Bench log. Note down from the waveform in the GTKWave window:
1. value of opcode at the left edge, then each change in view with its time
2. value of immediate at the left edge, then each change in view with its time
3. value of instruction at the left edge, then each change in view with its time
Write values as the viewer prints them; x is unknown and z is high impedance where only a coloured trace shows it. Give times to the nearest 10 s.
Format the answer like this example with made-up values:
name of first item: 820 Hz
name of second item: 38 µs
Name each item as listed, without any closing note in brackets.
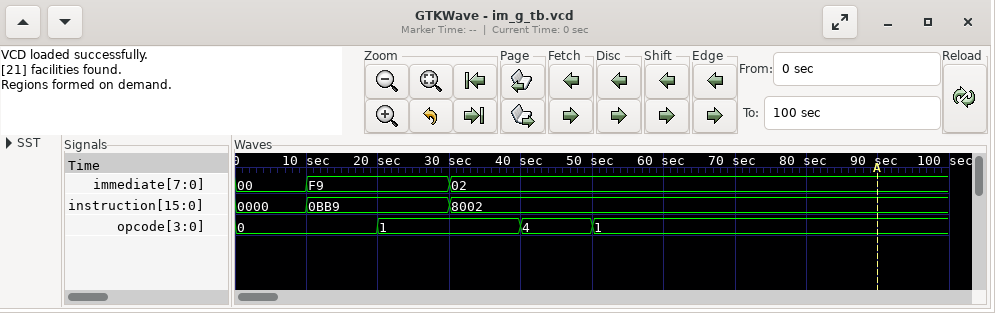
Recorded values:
value of opcode at the left edge, then each change in view with its time: 0, 1 at 20 s, 4 at 40 s, 1 at 50 s
value of immediate at the left edge, then each change in view with its time: 00, F9 at 10 s, 02 at 30 s
value of instruction at the left edge, then each change in view with its time: 0000, 0BB9 at 10 s, 8002 at 30 s
